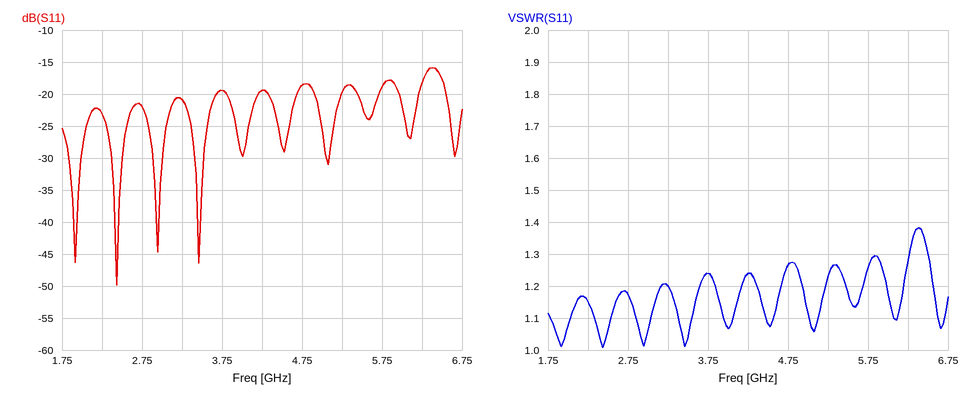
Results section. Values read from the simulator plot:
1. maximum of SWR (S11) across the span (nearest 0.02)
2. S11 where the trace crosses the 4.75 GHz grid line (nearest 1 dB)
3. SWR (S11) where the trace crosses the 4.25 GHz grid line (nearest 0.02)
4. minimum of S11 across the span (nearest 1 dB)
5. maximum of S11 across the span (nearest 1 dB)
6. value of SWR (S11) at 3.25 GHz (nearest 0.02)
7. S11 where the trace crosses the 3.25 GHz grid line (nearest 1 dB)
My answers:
1.38
-19 dB
1.24
-50 dB
-16 dB
1.20
-21 dB
